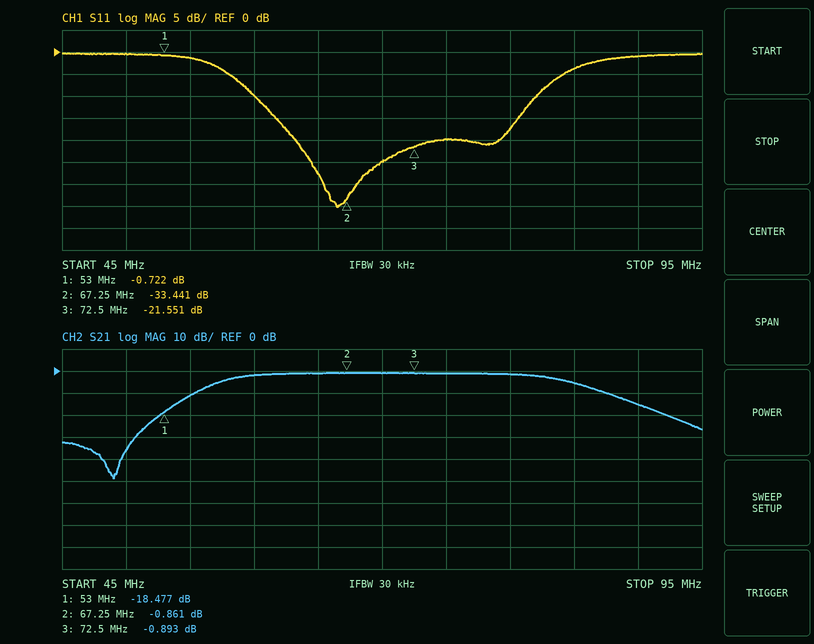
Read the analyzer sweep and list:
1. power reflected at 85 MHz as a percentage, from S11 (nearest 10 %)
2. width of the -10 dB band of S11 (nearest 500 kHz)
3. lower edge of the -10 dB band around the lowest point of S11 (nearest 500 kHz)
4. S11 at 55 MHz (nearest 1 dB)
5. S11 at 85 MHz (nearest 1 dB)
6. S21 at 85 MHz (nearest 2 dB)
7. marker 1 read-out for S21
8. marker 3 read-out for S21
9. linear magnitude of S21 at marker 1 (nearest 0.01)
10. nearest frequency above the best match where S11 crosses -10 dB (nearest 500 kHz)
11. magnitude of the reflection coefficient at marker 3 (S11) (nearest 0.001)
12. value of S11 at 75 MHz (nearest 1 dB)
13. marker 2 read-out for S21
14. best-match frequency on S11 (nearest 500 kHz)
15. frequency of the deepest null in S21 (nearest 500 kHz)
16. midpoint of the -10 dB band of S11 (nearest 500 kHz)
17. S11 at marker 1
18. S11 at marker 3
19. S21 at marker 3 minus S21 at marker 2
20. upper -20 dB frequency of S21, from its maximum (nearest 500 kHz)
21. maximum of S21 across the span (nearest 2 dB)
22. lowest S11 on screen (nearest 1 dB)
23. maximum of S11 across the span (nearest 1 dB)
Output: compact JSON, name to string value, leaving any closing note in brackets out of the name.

{"power reflected at 85 MHz as a percentage, from S11": "40 %", "width of the -10 dB band of S11": "22.0 MHz", "lower edge of the -10 dB band around the lowest point of S11": "60.0 MHz", "S11 at 55 MHz": "-1 dB", "S11 at 85 MHz": "-4 dB", "S21 at 85 MHz": "-6 dB", "marker 1 read-out for S21": "-18.477 dB", "marker 3 read-out for S21": "-0.893 dB", "linear magnitude of S21 at marker 1": "0.12", "nearest frequency above the best match where S11 crosses -10 dB": "82.0 MHz", "magnitude of the reflection coefficient at marker 3 (S11)": "0.084", "value of S11 at 75 MHz": "-20 dB", "marker 2 read-out for S21": "-0.861 dB", "best-match frequency on S11": "66.5 MHz", "frequency of the deepest null in S21": "49.0 MHz", "midpoint of the -10 dB band of S11": "71.0 MHz", "S11 at marker 1": "-0.722 dB", "S11 at marker 3": "-21.551 dB", "S21 at marker 3 minus S21 at marker 2": "-0.032 dB", "upper -20 dB frequency of S21, from its maximum": "92.5 MHz", "maximum of S21 across the span": "0 dB", "lowest S11 on screen": "-35 dB", "maximum of S11 across the span": "0 dB"}
